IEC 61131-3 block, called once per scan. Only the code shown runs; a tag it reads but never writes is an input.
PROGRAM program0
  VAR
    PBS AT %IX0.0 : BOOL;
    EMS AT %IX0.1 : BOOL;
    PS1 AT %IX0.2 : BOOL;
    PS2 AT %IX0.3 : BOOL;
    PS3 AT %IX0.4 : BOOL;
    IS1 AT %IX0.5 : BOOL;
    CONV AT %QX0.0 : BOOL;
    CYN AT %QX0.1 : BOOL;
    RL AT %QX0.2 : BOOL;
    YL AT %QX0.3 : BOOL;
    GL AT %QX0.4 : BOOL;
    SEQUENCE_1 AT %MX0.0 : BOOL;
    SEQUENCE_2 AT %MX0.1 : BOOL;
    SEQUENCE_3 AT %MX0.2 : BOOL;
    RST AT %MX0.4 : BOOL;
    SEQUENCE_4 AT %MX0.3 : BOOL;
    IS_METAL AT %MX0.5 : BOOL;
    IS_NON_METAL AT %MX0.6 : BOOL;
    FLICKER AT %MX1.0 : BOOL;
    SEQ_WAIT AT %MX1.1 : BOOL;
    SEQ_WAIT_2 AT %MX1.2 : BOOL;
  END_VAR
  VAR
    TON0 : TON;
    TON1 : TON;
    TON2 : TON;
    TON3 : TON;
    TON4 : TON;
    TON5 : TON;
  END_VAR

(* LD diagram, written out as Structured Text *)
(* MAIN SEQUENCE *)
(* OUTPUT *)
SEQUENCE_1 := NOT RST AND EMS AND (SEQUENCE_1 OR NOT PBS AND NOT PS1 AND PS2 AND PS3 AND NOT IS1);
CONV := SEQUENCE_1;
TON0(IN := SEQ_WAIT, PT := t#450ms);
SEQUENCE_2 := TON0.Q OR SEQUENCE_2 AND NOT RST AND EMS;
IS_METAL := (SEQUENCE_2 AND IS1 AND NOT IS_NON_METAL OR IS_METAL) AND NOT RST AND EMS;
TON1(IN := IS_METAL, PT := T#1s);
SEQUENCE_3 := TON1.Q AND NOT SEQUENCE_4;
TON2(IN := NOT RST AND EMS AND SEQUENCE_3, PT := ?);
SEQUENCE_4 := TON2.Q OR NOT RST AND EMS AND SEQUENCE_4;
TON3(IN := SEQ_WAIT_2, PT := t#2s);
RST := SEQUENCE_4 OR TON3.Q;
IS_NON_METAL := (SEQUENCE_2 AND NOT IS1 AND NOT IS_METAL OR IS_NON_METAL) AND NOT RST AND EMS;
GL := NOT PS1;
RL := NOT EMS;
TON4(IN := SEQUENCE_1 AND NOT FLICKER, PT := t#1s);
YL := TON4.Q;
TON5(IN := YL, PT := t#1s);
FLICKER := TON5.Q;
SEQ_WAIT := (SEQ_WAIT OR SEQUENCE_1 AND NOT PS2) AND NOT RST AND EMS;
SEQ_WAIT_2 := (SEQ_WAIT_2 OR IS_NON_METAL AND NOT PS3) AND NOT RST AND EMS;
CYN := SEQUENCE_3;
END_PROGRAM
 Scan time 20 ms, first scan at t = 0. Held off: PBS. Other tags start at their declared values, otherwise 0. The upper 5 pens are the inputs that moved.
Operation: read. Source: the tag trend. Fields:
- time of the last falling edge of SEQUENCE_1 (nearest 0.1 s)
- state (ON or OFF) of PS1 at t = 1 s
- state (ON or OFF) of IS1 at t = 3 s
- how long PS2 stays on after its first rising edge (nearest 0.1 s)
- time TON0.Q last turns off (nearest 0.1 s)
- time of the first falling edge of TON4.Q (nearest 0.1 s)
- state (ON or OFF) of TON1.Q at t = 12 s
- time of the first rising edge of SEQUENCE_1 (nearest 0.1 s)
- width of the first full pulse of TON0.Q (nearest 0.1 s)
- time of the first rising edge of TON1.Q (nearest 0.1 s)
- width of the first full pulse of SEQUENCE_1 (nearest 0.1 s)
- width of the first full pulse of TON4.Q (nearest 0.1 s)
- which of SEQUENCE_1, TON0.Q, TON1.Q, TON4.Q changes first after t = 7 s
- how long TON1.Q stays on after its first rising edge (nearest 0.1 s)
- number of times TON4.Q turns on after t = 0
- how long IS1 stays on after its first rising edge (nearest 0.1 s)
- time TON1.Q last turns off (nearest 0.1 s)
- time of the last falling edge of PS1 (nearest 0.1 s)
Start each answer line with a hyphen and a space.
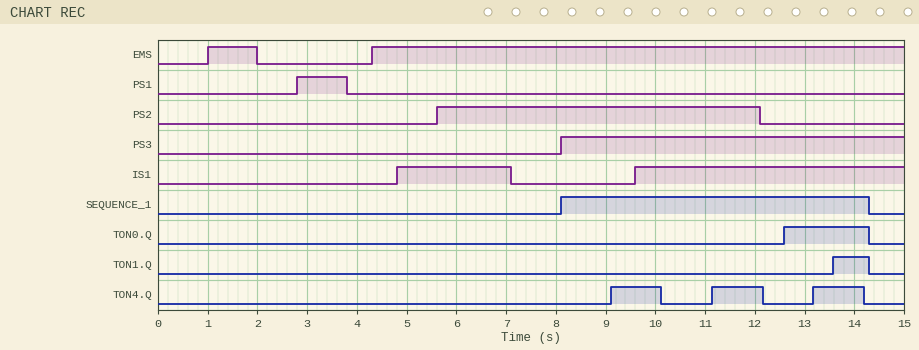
- 14.3 s
- OFF
- OFF
- 6.5 s
- 14.3 s
- 10.1 s
- OFF
- 8.1 s
- 1.7 s
- 13.6 s
- 6.2 s
- 1.0 s
- SEQUENCE_1
- 0.7 s
- 3
- 2.3 s
- 14.3 s
- 3.8 s
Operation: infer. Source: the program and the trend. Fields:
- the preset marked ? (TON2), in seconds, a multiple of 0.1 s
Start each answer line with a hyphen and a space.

- 0.7 s
